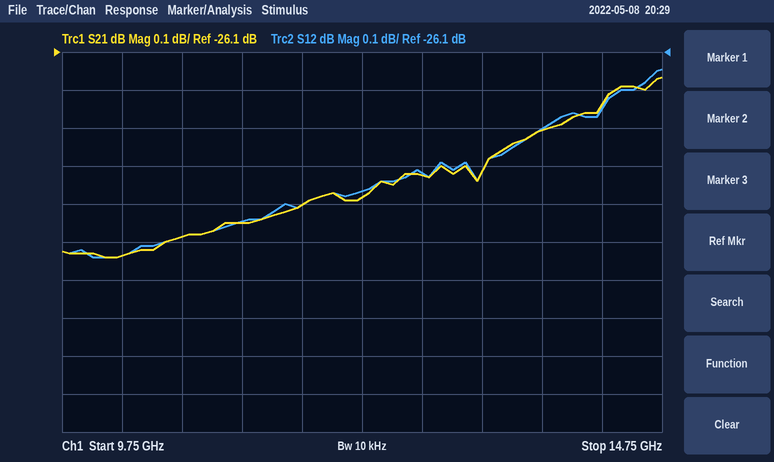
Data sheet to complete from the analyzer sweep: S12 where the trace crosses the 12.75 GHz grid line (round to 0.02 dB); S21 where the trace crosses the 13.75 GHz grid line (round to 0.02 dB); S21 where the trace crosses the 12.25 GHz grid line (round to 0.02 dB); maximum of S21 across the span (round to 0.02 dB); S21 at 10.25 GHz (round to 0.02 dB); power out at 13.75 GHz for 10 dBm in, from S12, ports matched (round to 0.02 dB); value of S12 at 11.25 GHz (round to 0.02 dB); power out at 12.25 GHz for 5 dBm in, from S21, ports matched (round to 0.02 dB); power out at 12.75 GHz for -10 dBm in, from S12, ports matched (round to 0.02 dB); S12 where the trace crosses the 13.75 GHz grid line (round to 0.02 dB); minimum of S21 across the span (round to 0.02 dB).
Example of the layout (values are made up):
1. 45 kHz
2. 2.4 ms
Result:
1. -26.42 dB
2. -26.30 dB
3. -26.48 dB
4. -26.16 dB
5. -26.64 dB
6. -16.30 dBm
7. -26.54 dB
8. -21.48 dBm
9. -36.42 dBm
10. -26.30 dB
11. -26.64 dB
